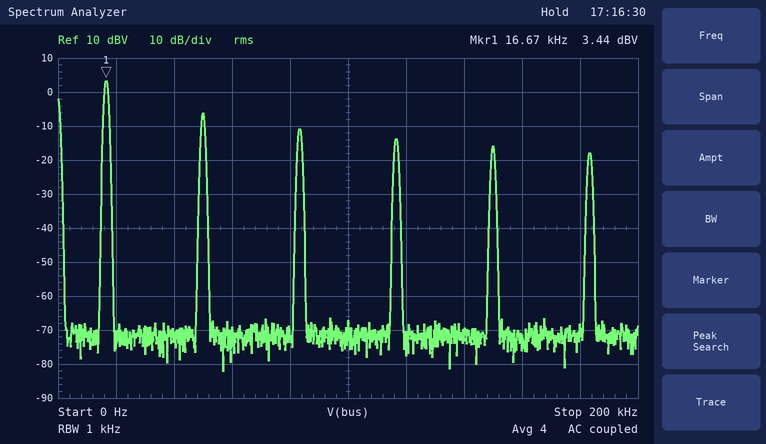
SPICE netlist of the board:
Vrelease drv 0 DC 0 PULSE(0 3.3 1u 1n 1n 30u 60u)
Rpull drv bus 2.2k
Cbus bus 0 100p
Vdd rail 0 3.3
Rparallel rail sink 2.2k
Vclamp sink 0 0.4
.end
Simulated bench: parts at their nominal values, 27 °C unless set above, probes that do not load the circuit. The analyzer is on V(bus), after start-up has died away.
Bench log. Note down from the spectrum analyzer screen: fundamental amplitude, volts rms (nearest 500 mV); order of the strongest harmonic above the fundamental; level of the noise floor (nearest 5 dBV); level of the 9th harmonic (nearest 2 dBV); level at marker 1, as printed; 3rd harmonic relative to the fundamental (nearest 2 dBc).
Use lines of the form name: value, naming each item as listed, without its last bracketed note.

fundamental amplitude, volts rms: 1.5 V
order of the strongest harmonic above the fundamental: 3
level of the noise floor: -70 dBV
level of the 9th harmonic: -16 dBV
level at marker 1, as printed: 3.44 dBV
3rd harmonic relative to the fundamental: -10 dBc
